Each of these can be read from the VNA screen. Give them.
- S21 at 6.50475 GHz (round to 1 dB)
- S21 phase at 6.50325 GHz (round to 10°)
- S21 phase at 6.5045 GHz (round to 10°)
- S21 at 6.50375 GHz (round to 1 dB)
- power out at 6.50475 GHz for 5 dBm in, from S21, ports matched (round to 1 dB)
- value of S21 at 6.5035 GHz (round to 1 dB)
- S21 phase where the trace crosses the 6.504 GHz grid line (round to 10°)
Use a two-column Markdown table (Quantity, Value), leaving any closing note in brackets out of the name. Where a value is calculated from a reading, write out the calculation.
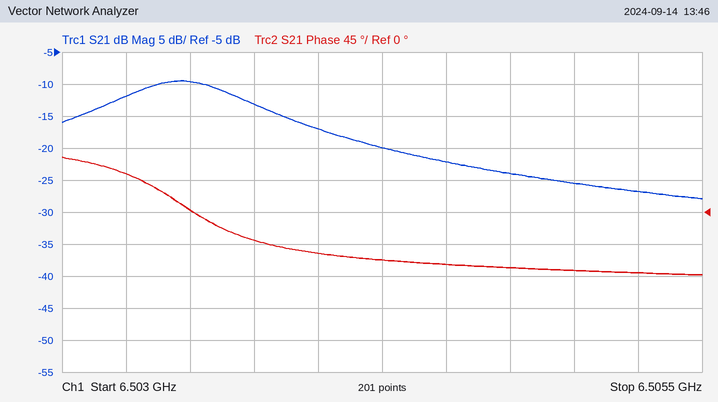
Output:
| Quantity | Value |
|---|---|
| S21 at 6.50475 GHz | -24 dB |
| S21 phase at 6.50325 GHz | 50° |
| S21 phase at 6.5045 GHz | -70° |
| S21 at 6.50375 GHz | -13 dB |
| power out at 6.50475 GHz for 5 dBm in, from S21, ports matched | 5 dBm + (-24 dB) = -19 dBm |
| value of S21 at 6.5035 GHz | -10 dB |
| S21 phase where the trace crosses the 6.504 GHz grid line | -60° |
